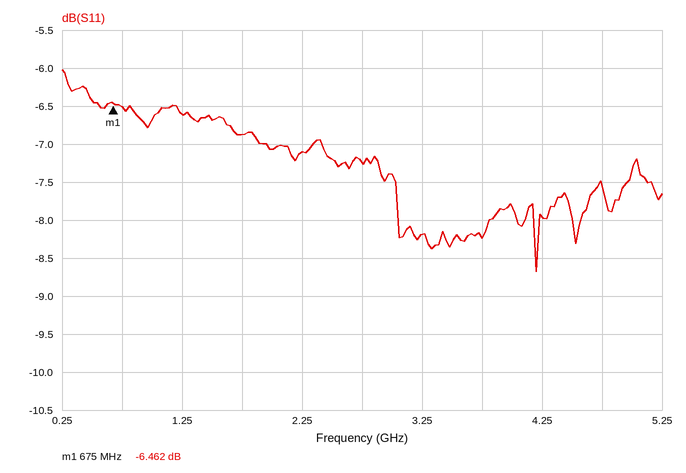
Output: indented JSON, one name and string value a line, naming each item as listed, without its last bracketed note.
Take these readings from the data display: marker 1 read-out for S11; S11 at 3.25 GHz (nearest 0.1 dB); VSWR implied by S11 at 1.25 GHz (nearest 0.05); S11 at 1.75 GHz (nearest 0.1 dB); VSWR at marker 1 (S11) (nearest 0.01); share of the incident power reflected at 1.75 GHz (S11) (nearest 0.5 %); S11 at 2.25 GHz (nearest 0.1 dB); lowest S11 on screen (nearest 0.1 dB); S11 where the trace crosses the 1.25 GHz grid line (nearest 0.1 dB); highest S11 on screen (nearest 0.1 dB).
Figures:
{
  "marker 1 read-out for S11": "-6.462 dB",
  "S11 at 3.25 GHz": "-8.2 dB",
  "VSWR implied by S11 at 1.25 GHz": "2.75",
  "S11 at 1.75 GHz": "-6.9 dB",
  "VSWR at marker 1 (S11)": "2.81",
  "share of the incident power reflected at 1.75 GHz (S11)": "20.5 %",
  "S11 at 2.25 GHz": "-7.1 dB",
  "lowest S11 on screen": "-8.7 dB",
  "S11 where the trace crosses the 1.25 GHz grid line": "-6.6 dB",
  "highest S11 on screen": "-6.0 dB"
}
